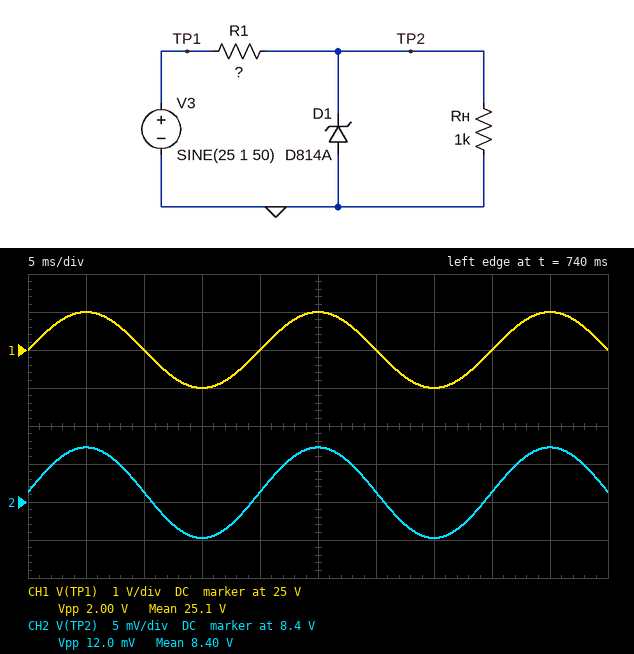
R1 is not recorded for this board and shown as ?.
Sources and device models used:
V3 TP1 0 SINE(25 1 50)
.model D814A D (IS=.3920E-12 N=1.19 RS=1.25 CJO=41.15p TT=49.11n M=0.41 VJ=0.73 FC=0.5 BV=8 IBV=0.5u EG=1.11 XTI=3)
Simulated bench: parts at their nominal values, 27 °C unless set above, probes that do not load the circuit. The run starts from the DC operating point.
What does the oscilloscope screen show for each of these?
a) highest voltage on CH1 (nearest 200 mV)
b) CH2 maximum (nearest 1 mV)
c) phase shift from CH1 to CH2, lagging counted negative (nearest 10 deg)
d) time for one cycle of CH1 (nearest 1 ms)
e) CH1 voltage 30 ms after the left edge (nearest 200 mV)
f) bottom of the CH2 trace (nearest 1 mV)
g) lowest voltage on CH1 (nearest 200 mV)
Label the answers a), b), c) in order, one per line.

a) 26.0 V
b) 8.407 V
c) 0 deg
d) 20 ms
e) 25.0 V
f) 8.395 V
g) 24.0 V
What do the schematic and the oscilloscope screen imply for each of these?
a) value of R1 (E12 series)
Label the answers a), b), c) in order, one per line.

a) 330 Ω
